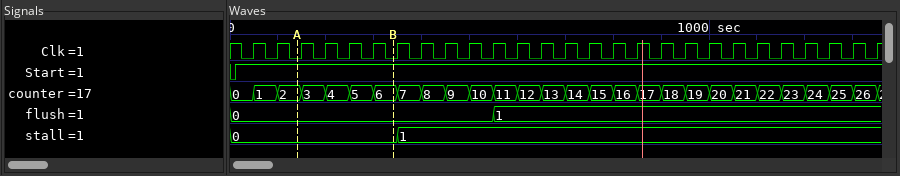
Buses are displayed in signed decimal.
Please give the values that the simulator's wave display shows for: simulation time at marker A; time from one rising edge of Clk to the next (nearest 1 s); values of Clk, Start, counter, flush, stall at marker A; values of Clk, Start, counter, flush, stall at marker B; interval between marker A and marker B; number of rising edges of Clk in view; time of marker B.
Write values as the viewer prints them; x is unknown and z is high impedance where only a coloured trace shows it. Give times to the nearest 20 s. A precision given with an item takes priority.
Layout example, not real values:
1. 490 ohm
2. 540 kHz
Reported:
1. 140 s
2. 50 s
3. Clk=0, Start=1, counter=2, flush=0, stall=0
4. Clk=0, Start=1, counter=6, flush=0, stall=0
5. 200 s
6. 27
7. 340 s
